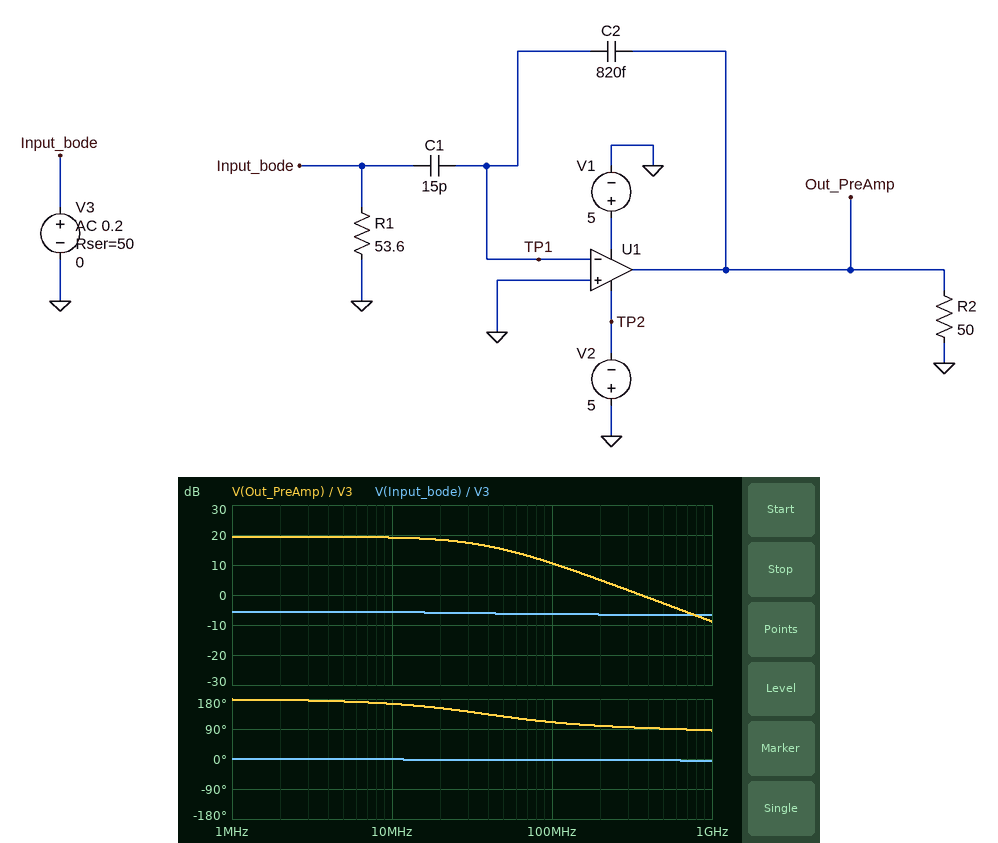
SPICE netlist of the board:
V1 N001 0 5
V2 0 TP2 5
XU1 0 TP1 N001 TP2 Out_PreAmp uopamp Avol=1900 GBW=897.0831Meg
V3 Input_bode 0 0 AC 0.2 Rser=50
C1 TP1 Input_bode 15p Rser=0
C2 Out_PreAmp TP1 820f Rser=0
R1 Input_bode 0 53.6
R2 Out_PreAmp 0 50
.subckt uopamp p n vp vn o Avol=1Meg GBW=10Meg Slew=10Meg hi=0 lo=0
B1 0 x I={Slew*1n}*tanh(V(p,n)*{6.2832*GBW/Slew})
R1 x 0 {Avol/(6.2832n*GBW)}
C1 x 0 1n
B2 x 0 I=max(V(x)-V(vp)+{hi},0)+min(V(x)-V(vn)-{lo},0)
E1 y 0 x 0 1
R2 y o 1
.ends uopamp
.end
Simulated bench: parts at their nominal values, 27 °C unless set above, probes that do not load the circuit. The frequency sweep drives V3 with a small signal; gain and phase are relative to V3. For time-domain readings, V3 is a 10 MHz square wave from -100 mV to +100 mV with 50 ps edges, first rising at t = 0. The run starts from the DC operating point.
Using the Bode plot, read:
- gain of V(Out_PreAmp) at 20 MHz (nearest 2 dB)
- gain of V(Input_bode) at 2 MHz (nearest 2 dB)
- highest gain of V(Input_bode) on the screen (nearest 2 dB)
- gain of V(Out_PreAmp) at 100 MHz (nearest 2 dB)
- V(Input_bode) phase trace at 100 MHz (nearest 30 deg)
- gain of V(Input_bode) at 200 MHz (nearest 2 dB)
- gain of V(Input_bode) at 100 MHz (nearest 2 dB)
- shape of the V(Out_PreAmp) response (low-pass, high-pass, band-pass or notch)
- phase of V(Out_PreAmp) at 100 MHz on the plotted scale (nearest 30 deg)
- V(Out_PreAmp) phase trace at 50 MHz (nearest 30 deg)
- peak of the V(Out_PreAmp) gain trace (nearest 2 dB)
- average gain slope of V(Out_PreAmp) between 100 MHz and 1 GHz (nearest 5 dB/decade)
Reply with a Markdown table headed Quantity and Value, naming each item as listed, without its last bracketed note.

| Quantity | Value |
|---|---|
| gain of V(Out_PreAmp) at 20 MHz | 18 dB |
| gain of V(Input_bode) at 2 MHz | -6 dB |
| highest gain of V(Input_bode) on the screen | -6 dB |
| gain of V(Out_PreAmp) at 100 MHz | 10 dB |
| V(Input_bode) phase trace at 100 MHz | 0 deg |
| gain of V(Input_bode) at 200 MHz | -6 dB |
| gain of V(Input_bode) at 100 MHz | -6 dB |
| shape of the V(Out_PreAmp) response | low-pass |
| phase of V(Out_PreAmp) at 100 MHz on the plotted scale | 120 deg |
| V(Out_PreAmp) phase trace at 50 MHz | 120 deg |
| peak of the V(Out_PreAmp) gain trace | 20 dB |
| average gain slope of V(Out_PreAmp) between 100 MHz and 1 GHz | -20 dB/decade |
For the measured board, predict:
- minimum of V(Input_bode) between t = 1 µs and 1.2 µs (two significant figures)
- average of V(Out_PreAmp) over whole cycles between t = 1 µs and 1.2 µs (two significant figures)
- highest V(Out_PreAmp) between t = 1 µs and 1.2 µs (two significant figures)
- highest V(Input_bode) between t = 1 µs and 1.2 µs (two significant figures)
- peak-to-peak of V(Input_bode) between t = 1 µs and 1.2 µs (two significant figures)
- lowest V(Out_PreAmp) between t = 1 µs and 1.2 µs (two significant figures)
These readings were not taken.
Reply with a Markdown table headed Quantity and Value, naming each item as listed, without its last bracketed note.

| Quantity | Value |
|---|---|
| minimum of V(Input_bode) between t = 1 µs and 1.2 µs | -52 mV |
| average of V(Out_PreAmp) over whole cycles between t = 1 µs and 1.2 µs | -220 mV |
| highest V(Out_PreAmp) between t = 1 µs and 1.2 µs | -2.7 mV |
| highest V(Input_bode) between t = 1 µs and 1.2 µs | 52 mV |
| peak-to-peak of V(Input_bode) between t = 1 µs and 1.2 µs | 100 mV |
| lowest V(Out_PreAmp) between t = 1 µs and 1.2 µs | -460 mV |
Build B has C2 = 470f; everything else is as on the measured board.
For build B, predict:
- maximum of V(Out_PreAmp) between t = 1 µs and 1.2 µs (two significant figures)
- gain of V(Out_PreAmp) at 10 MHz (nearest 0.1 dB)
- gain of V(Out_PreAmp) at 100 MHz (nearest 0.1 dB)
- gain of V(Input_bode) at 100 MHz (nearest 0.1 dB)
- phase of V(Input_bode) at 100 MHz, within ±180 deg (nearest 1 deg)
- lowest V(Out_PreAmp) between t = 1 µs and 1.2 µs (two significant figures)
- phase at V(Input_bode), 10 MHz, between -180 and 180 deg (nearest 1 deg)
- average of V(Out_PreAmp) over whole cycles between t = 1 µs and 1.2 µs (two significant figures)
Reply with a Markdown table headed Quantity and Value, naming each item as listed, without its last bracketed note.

| Quantity | Value |
|---|---|
| maximum of V(Out_PreAmp) between t = 1 µs and 1.2 µs | -12 mV |
| gain of V(Out_PreAmp) at 10 MHz | 23.6 dB |
| gain of V(Out_PreAmp) at 100 MHz | 12.1 dB |
| gain of V(Input_bode) at 100 MHz | -6.2 dB |
| phase of V(Input_bode) at 100 MHz, within ±180 deg | -1 deg |
| lowest V(Out_PreAmp) between t = 1 µs and 1.2 µs | -470 mV |
| phase at V(Input_bode), 10 MHz, between -180 and 180 deg | -1 deg |
| average of V(Out_PreAmp) over whole cycles between t = 1 µs and 1.2 µs | -230 mV |
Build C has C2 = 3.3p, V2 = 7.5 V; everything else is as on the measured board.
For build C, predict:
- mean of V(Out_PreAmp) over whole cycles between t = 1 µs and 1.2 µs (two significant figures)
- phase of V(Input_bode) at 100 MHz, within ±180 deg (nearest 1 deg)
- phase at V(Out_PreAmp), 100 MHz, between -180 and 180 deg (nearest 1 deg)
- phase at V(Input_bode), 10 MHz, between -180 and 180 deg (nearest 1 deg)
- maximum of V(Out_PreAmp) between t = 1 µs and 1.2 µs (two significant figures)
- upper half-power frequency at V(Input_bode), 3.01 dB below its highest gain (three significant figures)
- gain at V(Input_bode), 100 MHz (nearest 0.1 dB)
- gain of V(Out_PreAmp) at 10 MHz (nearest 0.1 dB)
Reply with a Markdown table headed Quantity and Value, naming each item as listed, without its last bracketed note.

| Quantity | Value |
|---|---|
| mean of V(Out_PreAmp) over whole cycles between t = 1 µs and 1.2 µs | -210 mV |
| phase of V(Input_bode) at 100 MHz, within ±180 deg | -10 deg |
| phase at V(Out_PreAmp), 100 MHz, between -180 and 180 deg | 138 deg |
| phase at V(Input_bode), 10 MHz, between -180 and 180 deg | -1 deg |
| maximum of V(Out_PreAmp) between t = 1 µs and 1.2 µs | 2.3 mV |
| upper half-power frequency at V(Input_bode), 3.01 dB below its highest gain | 1.06 GHz |
| gain at V(Input_bode), 100 MHz | -6.6 dB |
| gain of V(Out_PreAmp) at 10 MHz | 7.4 dB |
